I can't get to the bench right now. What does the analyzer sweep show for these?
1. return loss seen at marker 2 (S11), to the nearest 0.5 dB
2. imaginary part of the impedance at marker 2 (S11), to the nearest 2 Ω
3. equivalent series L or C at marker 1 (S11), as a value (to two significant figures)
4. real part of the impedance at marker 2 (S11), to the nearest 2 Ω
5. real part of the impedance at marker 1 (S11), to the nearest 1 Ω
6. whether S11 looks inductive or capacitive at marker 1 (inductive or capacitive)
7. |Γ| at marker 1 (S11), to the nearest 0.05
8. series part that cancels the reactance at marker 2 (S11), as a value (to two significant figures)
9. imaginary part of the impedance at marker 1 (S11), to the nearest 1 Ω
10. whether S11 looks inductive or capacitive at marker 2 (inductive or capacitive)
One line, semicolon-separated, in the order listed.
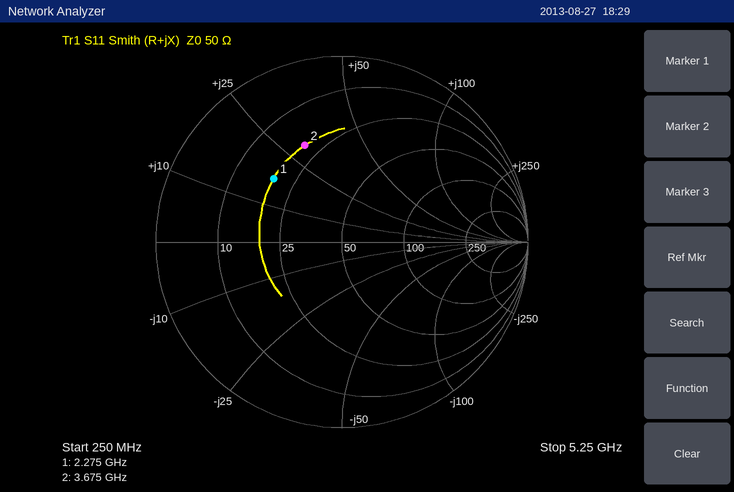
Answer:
5.0 dB; +30 Ω; 1.2 nH; 20 Ω; 19 Ω; inductive; 0.50; 1.4 pF; +17 Ω; inductive
